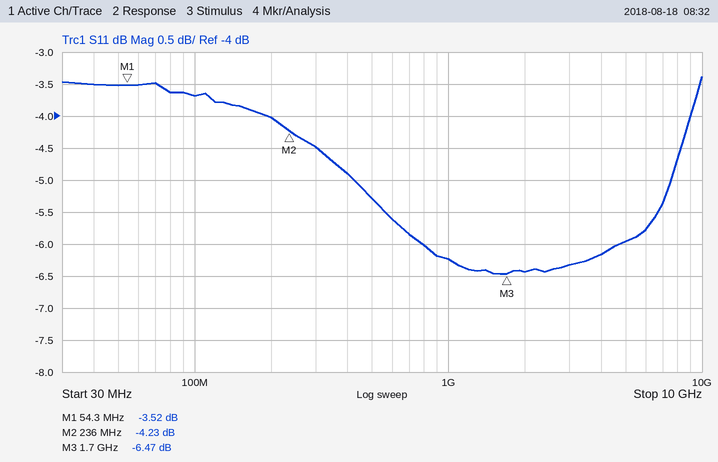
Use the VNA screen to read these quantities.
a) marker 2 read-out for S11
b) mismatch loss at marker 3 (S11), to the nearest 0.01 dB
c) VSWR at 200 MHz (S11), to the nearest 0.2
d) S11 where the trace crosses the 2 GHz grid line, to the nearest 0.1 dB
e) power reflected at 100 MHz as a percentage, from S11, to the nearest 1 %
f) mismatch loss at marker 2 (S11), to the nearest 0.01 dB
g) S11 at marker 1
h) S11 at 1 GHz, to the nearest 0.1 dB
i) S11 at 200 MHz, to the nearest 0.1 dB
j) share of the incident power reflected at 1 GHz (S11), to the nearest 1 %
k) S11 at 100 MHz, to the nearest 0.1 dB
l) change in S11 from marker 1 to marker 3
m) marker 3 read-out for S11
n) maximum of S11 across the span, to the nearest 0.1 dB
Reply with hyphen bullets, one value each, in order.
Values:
- -4.23 dB
- 1.11 dB
- 4.4
- -6.4 dB
- 43 %
- 2.06 dB
- -3.52 dB
- -6.2 dB
- -4.0 dB
- 24 %
- -3.7 dB
- -2.95 dB
- -6.47 dB
- -3.4 dB
